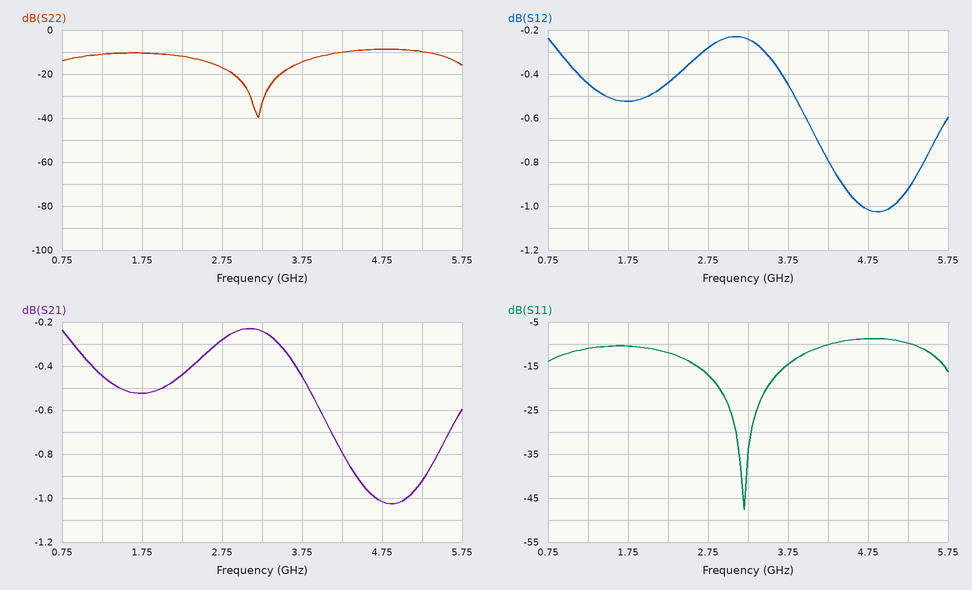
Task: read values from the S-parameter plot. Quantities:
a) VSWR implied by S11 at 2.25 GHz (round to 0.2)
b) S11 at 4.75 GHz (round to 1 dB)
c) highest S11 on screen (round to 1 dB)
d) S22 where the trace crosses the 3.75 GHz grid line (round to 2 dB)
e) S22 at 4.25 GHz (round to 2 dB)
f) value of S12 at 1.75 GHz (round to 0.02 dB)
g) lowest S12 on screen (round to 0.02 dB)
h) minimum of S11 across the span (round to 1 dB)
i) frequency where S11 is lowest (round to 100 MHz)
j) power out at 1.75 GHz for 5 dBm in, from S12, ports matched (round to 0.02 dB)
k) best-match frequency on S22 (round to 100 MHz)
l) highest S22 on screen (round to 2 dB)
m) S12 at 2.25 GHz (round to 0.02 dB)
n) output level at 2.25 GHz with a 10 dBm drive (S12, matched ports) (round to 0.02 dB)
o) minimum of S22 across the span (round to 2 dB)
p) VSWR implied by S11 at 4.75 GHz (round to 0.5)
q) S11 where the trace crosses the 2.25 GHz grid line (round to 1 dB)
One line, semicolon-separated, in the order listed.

1.6; -9 dB; -9 dB; -14 dB; -10 dB; -0.52 dB; -1.02 dB; -48 dB; 3.2 GHz; 4.48 dBm; 3.2 GHz; -8 dB; -0.44 dB; 9.56 dBm; -40 dB; 2.0; -12 dB
